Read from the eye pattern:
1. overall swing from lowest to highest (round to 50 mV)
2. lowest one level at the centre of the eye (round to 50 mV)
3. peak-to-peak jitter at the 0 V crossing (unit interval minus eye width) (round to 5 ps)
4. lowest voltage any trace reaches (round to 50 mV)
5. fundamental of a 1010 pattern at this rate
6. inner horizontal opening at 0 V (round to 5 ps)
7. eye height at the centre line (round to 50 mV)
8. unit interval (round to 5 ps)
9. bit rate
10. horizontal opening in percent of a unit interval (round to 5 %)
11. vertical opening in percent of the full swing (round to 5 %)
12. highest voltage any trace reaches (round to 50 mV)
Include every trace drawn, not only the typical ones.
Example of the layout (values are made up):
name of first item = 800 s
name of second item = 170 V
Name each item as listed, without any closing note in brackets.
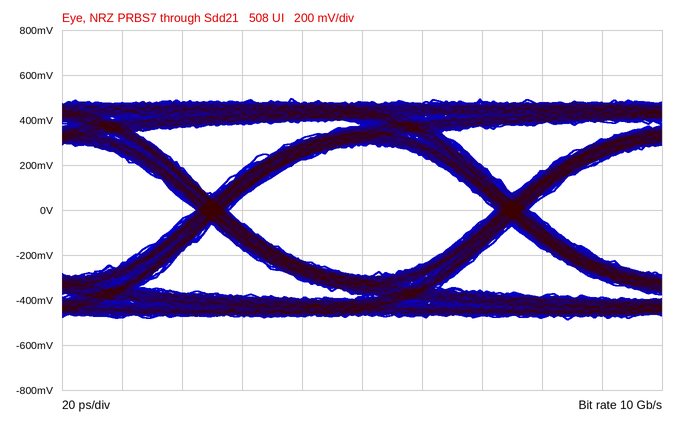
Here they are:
overall swing from lowest to highest = 1.00 V
lowest one level at the centre of the eye = 300 mV
peak-to-peak jitter at the 0 V crossing (unit interval minus eye width) = 10 ps
lowest voltage any trace reaches = -500 mV
fundamental of a 1010 pattern at this rate = 5 GHz
inner horizontal opening at 0 V = 90 ps
eye height at the centre line = 600 mV
unit interval = 100 ps
bit rate = 10 Gb/s
horizontal opening in percent of a unit interval = 90 %
vertical opening in percent of the full swing = 60 %
highest voltage any trace reaches = 500 mV
